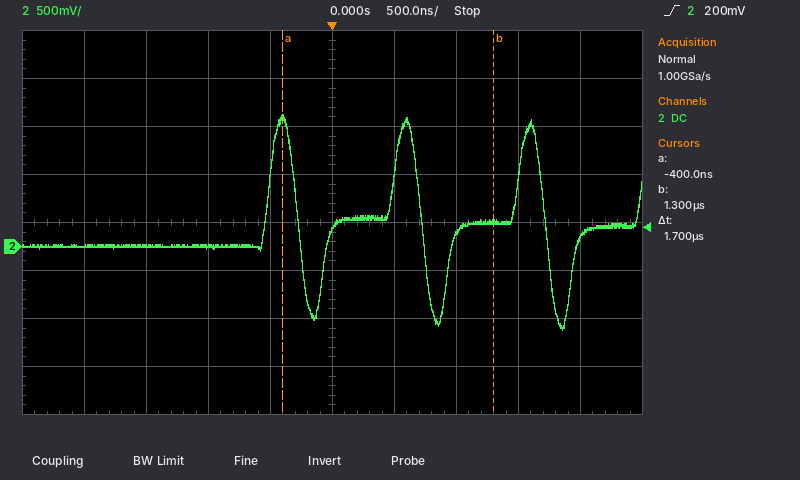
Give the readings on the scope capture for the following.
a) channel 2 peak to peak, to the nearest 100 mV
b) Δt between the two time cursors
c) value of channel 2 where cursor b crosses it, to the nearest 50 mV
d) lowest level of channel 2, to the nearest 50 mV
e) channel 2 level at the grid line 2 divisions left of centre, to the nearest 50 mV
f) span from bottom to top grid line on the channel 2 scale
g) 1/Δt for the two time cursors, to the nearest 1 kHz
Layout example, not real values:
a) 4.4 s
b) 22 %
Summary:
a) 2.20 V
b) 1.7 µs
c) 250 mV
d) -850 mV
e) 0 mV
f) 4 V
g) 588 kHz
